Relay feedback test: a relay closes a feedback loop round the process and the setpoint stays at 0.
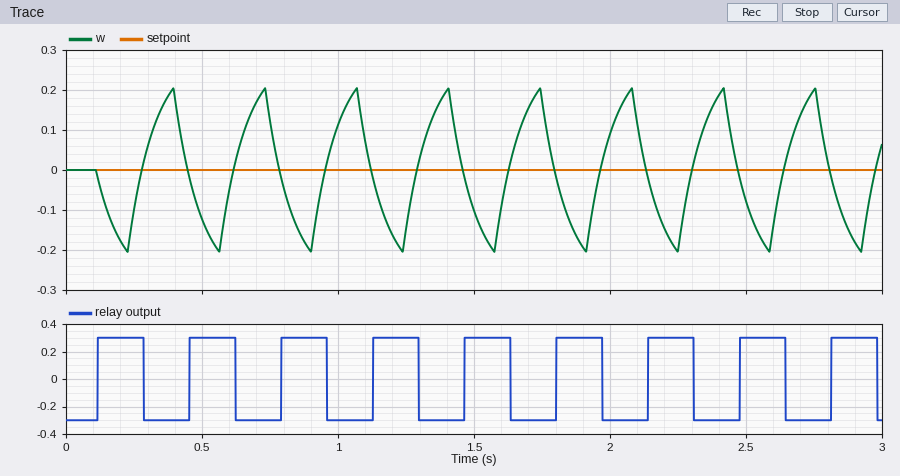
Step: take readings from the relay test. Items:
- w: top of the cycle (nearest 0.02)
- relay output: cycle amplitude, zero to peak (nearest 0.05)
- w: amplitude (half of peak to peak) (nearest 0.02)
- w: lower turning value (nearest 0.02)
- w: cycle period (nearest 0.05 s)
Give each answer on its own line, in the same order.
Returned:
0.20
0.30
0.20
-0.20
0.35 s
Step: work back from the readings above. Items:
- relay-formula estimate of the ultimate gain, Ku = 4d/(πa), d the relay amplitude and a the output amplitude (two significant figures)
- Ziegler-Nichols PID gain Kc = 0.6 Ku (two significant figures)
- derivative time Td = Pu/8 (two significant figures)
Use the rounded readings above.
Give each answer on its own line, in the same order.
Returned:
1.9
1.1
0.044 s
